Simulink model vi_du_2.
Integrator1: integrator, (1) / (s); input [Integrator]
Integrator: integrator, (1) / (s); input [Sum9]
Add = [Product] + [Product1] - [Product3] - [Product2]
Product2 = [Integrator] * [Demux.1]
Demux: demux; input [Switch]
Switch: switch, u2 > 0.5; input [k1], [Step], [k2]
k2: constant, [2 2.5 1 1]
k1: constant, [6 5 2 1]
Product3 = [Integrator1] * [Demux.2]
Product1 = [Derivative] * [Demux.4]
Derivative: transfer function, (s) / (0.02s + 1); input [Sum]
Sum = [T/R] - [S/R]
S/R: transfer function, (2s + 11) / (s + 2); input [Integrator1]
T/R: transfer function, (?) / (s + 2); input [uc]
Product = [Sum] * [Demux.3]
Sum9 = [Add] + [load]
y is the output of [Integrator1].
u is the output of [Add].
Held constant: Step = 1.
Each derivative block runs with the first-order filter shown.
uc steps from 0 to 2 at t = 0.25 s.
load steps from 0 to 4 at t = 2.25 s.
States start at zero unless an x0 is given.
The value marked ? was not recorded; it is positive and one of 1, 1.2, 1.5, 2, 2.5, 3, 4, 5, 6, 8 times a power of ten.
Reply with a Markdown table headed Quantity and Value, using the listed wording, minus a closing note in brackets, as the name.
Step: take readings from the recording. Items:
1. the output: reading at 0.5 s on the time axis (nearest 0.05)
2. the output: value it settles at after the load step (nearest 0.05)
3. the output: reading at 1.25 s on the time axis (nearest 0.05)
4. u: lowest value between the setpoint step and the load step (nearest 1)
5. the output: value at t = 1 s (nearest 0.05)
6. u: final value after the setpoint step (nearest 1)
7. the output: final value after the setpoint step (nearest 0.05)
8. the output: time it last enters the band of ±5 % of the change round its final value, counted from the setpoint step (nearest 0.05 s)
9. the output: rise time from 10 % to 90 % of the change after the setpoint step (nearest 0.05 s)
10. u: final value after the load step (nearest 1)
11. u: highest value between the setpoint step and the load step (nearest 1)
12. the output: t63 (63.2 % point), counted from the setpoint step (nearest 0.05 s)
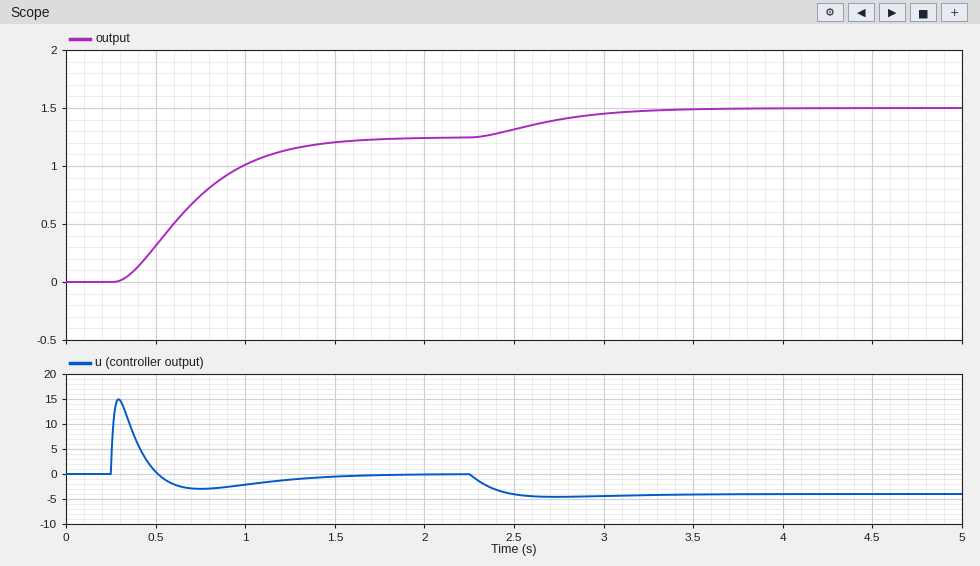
| Quantity | Value |
|---|---|
| the output: reading at 0.5 s on the time axis | 0.30 |
| the output: value it settles at after the load step | 1.50 |
| the output: reading at 1.25 s on the time axis | 1.15 |
| u: lowest value between the setpoint step and the load step | -3 |
| the output: value at t = 1 s | 1.00 |
| u: final value after the setpoint step | 0 |
| the output: final value after the setpoint step | 1.25 |
| the output: time it last enters the band of ±5 % of the change round its final value, counted from the setpoint step | 1.15 s |
| the output: rise time from 10 % to 90 % of the change after the setpoint step | 0.80 s |
| u: final value after the load step | -4 |
| u: highest value between the setpoint step and the load step | 15 |
| the output: t63 (63.2 % point), counted from the setpoint step | 0.55 s |
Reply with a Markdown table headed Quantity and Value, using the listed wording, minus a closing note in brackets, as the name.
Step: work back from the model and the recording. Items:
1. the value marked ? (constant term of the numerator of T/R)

| Quantity | Value |
|---|---|
| the value marked ? | 10 |
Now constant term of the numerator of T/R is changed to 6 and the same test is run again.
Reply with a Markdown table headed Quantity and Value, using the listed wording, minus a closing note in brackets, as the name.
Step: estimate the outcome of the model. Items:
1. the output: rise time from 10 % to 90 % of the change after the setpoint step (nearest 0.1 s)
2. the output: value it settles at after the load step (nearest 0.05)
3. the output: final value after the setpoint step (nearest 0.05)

| Quantity | Value |
|---|---|
| the output: rise time from 10 % to 90 % of the change after the setpoint step | 0.8 s |
| the output: value it settles at after the load step | 1.00 |
| the output: final value after the setpoint step | 0.75 |
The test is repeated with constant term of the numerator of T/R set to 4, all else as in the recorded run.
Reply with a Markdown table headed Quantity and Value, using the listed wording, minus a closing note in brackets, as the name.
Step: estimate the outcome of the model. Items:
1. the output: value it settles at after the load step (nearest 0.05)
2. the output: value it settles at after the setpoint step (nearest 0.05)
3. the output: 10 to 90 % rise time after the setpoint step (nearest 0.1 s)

| Quantity | Value |
|---|---|
| the output: value it settles at after the load step | 0.75 |
| the output: value it settles at after the setpoint step | 0.50 |
| the output: 10 to 90 % rise time after the setpoint step | 0.8 s |
